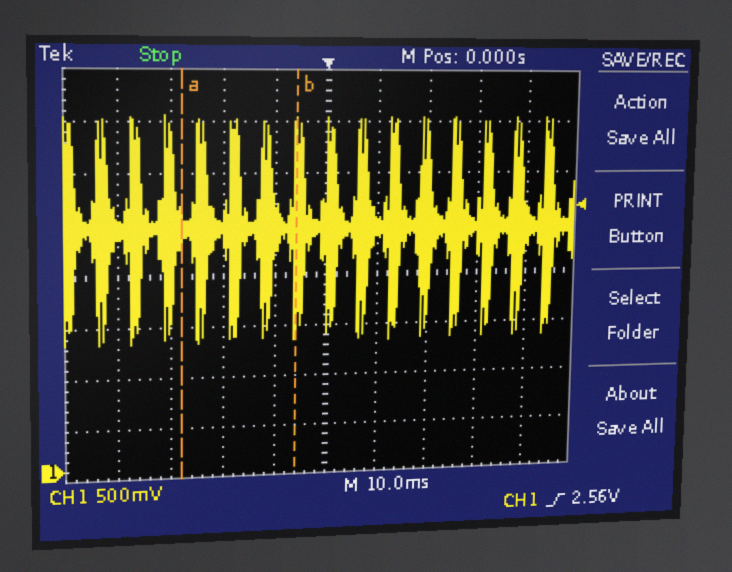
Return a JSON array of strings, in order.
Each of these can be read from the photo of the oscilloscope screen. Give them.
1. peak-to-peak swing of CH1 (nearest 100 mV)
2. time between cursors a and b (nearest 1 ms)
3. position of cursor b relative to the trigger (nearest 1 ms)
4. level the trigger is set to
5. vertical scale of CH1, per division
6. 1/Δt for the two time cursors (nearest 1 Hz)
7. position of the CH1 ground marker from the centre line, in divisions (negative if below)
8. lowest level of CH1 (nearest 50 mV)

["2.20 V", "22 ms", "-6 ms", "2.56 V", "500 mV", "45 Hz", "-3.8 div", "1.25 V"]
